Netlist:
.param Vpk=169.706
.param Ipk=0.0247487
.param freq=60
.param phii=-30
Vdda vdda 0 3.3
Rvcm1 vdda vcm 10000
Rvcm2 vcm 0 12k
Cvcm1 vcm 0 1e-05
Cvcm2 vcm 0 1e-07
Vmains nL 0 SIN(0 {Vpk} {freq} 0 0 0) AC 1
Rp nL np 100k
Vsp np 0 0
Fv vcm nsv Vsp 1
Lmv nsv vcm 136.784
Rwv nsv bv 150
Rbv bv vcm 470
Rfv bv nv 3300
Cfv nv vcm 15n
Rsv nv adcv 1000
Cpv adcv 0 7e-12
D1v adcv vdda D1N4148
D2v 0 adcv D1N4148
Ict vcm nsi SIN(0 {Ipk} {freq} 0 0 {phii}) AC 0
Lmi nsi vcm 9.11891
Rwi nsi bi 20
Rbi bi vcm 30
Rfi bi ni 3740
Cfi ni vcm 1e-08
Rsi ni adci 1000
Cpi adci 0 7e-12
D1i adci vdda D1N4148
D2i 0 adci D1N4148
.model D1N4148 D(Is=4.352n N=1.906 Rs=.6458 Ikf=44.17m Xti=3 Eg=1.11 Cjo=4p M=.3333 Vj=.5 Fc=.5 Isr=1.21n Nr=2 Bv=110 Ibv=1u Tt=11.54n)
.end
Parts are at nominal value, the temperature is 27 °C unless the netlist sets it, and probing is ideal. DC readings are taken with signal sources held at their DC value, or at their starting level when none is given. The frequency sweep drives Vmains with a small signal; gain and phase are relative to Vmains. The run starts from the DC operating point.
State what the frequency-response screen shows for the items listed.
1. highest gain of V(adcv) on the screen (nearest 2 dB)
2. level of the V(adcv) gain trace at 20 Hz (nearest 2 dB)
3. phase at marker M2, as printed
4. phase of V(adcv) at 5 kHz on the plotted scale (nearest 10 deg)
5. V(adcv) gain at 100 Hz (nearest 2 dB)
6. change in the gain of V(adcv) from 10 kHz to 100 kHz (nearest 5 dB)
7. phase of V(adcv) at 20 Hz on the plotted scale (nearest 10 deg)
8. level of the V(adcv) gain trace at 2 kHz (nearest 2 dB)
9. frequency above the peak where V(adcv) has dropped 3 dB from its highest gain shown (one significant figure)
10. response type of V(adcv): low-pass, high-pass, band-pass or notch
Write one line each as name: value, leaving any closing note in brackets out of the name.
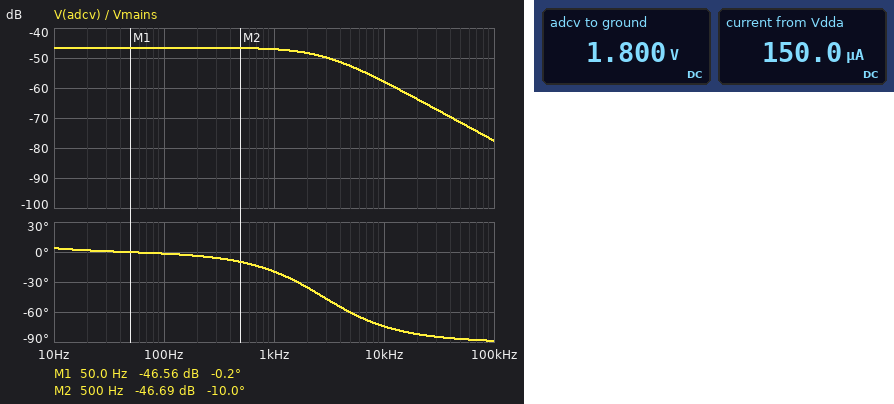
highest gain of V(adcv) on the screen: -46 dB
level of the V(adcv) gain trace at 20 Hz: -46 dB
phase at marker M2, as printed: -10.0 deg
phase of V(adcv) at 5 kHz on the plotted scale: -60 deg
V(adcv) gain at 100 Hz: -46 dB
change in the gain of V(adcv) from 10 kHz to 100 kHz: -20 dB
phase of V(adcv) at 20 Hz on the plotted scale: 0 deg
level of the V(adcv) gain trace at 2 kHz: -48 dB
frequency above the peak where V(adcv) has dropped 3 dB from its highest gain shown: 3 kHz
response type of V(adcv): low-pass, high-pass, band-pass or notch: low-pass
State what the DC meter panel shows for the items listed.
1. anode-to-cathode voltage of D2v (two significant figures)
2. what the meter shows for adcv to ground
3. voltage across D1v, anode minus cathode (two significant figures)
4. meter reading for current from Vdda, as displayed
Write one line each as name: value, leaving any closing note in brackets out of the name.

anode-to-cathode voltage of D2v: -1.8 V
what the meter shows for adcv to ground: 1.800 V
voltage across D1v, anode minus cathode: -1.5 V
meter reading for current from Vdda, as displayed: 150.0 µA
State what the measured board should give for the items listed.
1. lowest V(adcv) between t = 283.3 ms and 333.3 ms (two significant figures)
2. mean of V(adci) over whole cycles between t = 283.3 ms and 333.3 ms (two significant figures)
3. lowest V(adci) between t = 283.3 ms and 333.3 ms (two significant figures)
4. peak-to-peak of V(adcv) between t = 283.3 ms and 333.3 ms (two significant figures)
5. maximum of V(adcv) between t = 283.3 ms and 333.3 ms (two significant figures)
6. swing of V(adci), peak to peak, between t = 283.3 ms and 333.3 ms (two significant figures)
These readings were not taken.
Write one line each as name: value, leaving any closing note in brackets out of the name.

lowest V(adcv) between t = 283.3 ms and 333.3 ms: 1.0 V
mean of V(adci) over whole cycles between t = 283.3 ms and 333.3 ms: 1.9 V
lowest V(adci) between t = 283.3 ms and 333.3 ms: 1.1 V
peak-to-peak of V(adcv) between t = 283.3 ms and 333.3 ms: 1.6 V
maximum of V(adcv) between t = 283.3 ms and 333.3 ms: 2.6 V
swing of V(adci), peak to peak, between t = 283.3 ms and 333.3 ms: 1.5 V
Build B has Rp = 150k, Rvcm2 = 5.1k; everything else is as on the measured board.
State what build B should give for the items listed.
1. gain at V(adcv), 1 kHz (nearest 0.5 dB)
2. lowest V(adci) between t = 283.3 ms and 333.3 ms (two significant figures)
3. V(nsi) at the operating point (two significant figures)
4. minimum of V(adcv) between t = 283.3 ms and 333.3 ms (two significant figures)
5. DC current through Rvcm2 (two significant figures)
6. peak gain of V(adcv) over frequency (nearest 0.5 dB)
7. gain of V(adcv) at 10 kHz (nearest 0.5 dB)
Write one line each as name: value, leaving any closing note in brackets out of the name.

gain at V(adcv), 1 kHz: -50.5 dB
lowest V(adci) between t = 283.3 ms and 333.3 ms: 430 mV
V(nsi) at the operating point: 1.1 V
minimum of V(adcv) between t = 283.3 ms and 333.3 ms: 580 mV
DC current through Rvcm2: 220 µA
peak gain of V(adcv) over frequency: -50.0 dB
gain of V(adcv) at 10 kHz: -61.5 dB
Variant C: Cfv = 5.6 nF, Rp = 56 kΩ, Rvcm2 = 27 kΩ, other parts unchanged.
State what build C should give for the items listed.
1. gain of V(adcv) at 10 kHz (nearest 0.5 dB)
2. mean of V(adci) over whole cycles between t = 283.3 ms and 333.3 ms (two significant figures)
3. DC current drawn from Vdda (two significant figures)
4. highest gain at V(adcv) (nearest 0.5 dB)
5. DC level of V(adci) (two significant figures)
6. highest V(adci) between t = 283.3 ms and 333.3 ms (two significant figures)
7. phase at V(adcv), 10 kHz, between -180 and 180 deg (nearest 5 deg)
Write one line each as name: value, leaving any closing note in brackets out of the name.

gain of V(adcv) at 10 kHz: -46.0 dB
mean of V(adci) over whole cycles between t = 283.3 ms and 333.3 ms: 2.5 V
DC current drawn from Vdda: 89 µA
highest gain at V(adcv): -41.5 dB
DC level of V(adci): 2.4 V
highest V(adci) between t = 283.3 ms and 333.3 ms: 3.2 V
phase at V(adcv), 10 kHz, between -180 and 180 deg: -55 deg
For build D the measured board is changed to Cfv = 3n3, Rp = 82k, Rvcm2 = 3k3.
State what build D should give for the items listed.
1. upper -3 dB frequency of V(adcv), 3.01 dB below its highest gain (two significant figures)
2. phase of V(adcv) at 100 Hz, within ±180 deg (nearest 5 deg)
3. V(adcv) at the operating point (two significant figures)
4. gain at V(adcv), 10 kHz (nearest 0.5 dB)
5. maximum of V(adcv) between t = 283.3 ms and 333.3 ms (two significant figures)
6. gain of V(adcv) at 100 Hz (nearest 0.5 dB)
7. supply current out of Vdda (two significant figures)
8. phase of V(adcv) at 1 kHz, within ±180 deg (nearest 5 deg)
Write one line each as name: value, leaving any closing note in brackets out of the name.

upper -3 dB frequency of V(adcv), 3.01 dB below its highest gain: 13 kHz
phase of V(adcv) at 100 Hz, within ±180 deg: 0 deg
V(adcv) at the operating point: 820 mV
gain at V(adcv), 10 kHz: -47.0 dB
maximum of V(adcv) between t = 283.3 ms and 333.3 ms: 1.8 V
gain of V(adcv) at 100 Hz: -45.0 dB
supply current out of Vdda: 250 µA
phase of V(adcv) at 1 kHz, within ±180 deg: -5 deg
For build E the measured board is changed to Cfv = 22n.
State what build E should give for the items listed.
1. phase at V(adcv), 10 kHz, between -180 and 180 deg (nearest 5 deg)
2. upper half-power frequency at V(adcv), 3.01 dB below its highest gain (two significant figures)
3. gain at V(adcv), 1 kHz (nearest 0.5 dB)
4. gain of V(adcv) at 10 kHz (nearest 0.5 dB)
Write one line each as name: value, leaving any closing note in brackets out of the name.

phase at V(adcv), 10 kHz, between -180 and 180 deg: -80 deg
upper half-power frequency at V(adcv), 3.01 dB below its highest gain: 1.9 kHz
gain at V(adcv), 1 kHz: -47.5 dB
gain of V(adcv) at 10 kHz: -61.0 dB
